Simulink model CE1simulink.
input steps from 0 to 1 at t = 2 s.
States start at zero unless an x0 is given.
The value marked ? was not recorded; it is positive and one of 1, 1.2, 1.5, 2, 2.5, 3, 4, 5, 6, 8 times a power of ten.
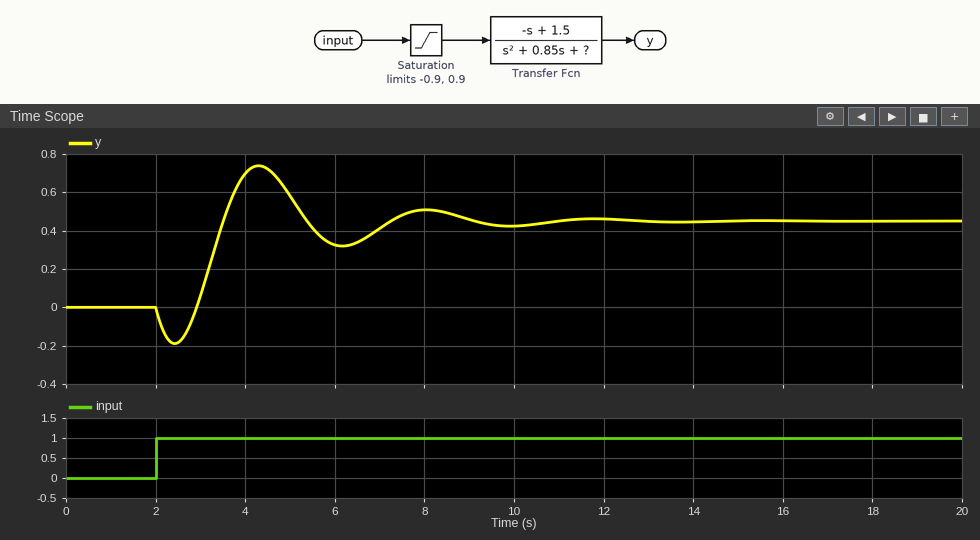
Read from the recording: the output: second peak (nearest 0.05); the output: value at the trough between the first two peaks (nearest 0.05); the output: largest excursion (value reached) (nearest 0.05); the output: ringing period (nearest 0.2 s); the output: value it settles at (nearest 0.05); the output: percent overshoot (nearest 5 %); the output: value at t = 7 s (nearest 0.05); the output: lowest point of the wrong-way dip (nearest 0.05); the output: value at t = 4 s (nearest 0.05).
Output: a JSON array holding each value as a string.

["0.50", "0.30", "0.75", "3.8 s", "0.45", "65 %", "0.40", "-0.20", "0.70"]
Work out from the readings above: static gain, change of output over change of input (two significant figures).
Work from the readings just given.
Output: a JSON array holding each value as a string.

["0.45"]
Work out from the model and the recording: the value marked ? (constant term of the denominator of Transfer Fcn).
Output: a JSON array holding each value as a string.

["3"]
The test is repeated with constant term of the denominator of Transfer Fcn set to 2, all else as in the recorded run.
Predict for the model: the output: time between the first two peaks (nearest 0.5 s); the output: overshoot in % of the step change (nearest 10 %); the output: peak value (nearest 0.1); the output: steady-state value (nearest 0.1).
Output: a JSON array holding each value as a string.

["4.5 s", "50 %", "1.0", "0.7"]
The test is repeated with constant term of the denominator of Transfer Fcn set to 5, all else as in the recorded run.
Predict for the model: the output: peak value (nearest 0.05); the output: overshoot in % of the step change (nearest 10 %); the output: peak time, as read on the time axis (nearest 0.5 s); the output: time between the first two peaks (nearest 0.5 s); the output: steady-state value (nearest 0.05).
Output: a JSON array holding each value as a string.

["0.50", "90 %", "4.0 s", "3.0 s", "0.25"]
